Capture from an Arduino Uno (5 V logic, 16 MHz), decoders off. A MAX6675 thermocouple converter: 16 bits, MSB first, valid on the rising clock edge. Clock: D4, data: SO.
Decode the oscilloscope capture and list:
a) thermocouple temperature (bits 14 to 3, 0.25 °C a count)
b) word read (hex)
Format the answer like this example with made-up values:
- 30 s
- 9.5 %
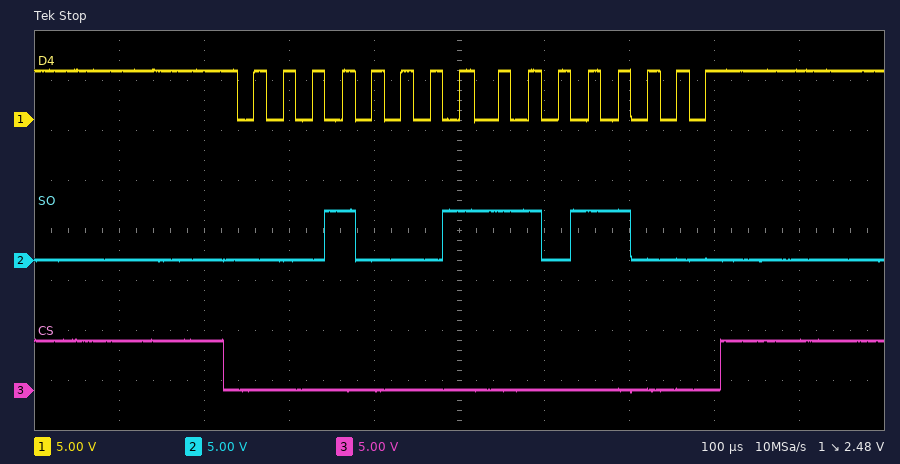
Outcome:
- 142.75 °C
- 0x11D8
